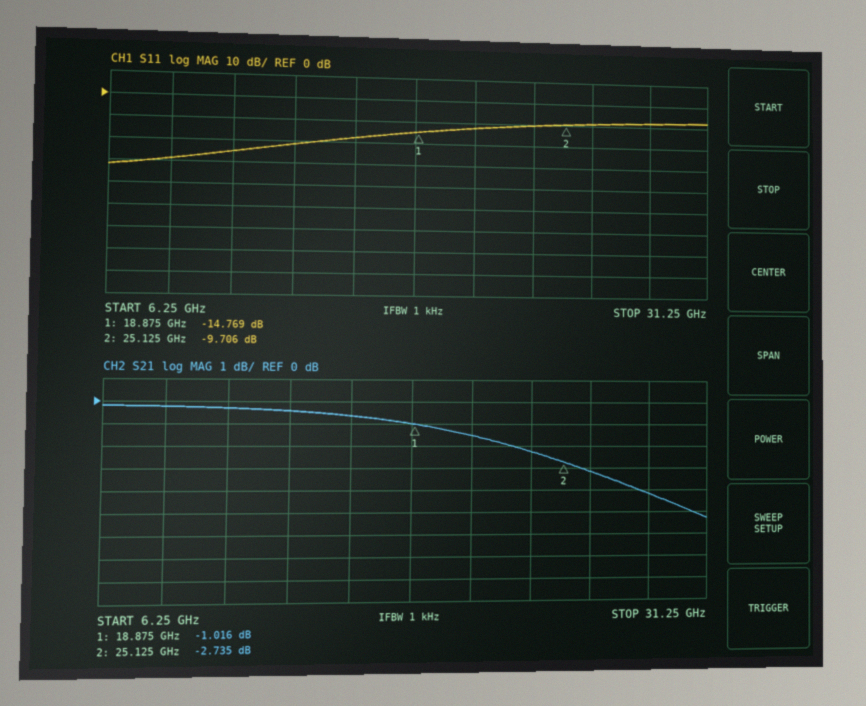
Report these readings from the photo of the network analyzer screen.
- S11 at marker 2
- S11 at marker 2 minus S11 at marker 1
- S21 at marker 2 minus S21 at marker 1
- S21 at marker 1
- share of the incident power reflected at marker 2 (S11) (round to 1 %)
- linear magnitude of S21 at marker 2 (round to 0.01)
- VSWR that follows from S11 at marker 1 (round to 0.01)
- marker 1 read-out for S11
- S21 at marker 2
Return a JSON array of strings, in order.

["-9.706 dB", "5.063 dB", "-1.719 dB", "-1.016 dB", "11 %", "0.73", "1.45", "-14.769 dB", "-2.735 dB"]
